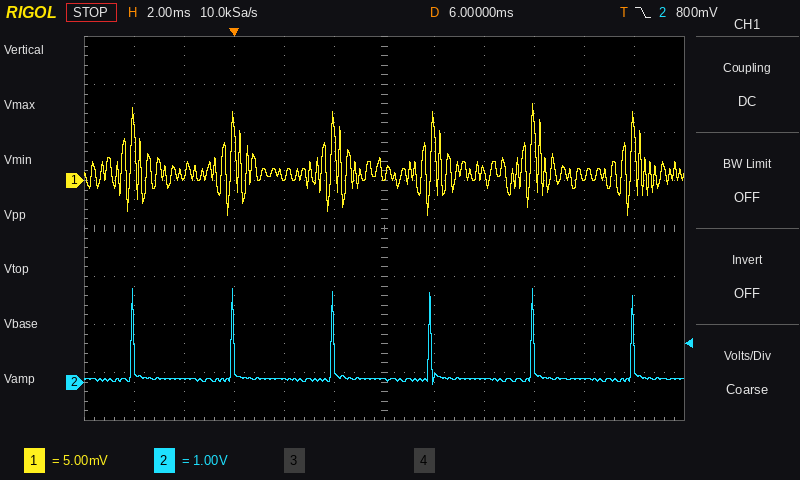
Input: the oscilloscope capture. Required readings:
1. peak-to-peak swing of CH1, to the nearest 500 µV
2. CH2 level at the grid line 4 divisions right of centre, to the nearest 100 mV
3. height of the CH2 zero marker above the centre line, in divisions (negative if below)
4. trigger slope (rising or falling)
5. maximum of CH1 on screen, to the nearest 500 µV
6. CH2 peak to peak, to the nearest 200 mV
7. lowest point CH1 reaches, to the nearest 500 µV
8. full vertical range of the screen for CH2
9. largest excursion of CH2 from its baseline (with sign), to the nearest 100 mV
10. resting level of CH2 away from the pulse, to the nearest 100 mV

11.5 mV
100 mV
-3.2 div
falling
8.0 mV
2.0 V
-3.5 mV
8 V
+1.9 V
100 mV
